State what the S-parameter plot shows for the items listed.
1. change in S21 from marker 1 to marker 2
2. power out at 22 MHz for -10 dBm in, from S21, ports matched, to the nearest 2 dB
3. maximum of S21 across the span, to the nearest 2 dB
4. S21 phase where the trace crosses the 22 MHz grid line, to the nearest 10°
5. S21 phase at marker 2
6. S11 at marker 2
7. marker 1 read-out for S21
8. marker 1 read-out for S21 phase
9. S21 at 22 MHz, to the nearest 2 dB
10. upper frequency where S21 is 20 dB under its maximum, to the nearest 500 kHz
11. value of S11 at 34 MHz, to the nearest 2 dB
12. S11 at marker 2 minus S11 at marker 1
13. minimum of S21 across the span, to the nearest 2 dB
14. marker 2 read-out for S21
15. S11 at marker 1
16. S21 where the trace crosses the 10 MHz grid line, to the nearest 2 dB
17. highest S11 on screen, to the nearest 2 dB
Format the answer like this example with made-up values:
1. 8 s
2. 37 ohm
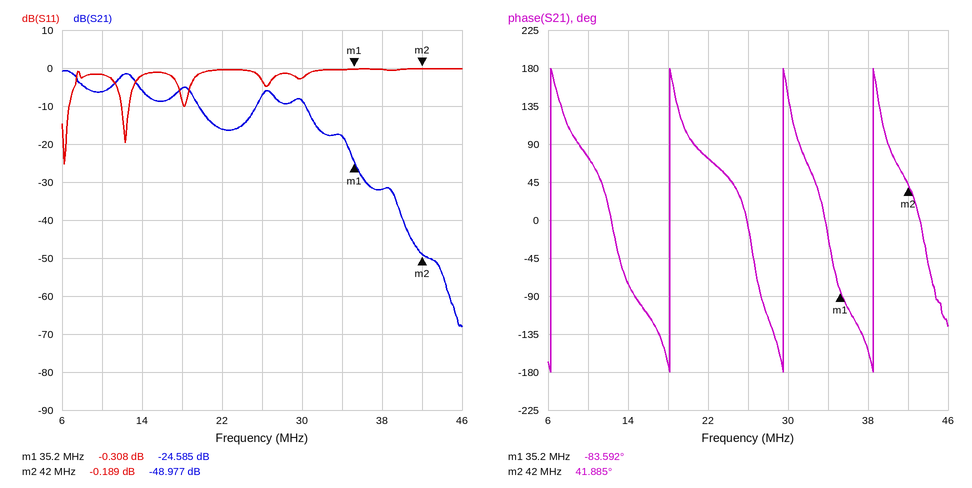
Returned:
1. -24.392 dB
2. -26 dBm
3. 0 dB
4. 70°
5. 41.885°
6. -0.189 dB
7. -24.585 dB
8. -83.592°
9. -16 dB
10. 34.5 MHz
11. 0 dB
12. 0.119 dB
13. -68 dB
14. -48.977 dB
15. -0.308 dB
16. -6 dB
17. 0 dB
